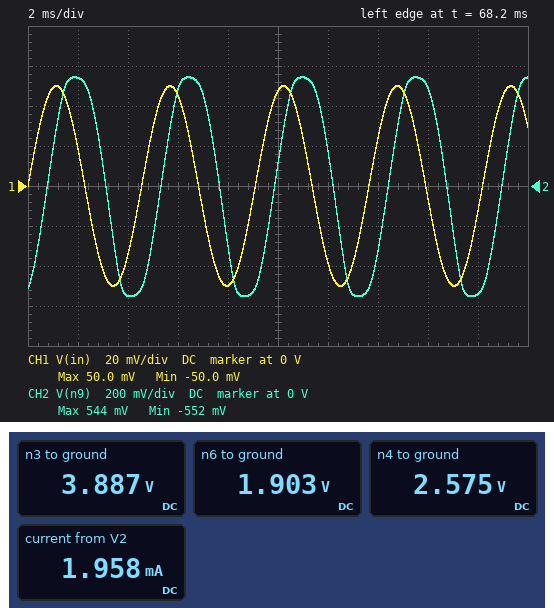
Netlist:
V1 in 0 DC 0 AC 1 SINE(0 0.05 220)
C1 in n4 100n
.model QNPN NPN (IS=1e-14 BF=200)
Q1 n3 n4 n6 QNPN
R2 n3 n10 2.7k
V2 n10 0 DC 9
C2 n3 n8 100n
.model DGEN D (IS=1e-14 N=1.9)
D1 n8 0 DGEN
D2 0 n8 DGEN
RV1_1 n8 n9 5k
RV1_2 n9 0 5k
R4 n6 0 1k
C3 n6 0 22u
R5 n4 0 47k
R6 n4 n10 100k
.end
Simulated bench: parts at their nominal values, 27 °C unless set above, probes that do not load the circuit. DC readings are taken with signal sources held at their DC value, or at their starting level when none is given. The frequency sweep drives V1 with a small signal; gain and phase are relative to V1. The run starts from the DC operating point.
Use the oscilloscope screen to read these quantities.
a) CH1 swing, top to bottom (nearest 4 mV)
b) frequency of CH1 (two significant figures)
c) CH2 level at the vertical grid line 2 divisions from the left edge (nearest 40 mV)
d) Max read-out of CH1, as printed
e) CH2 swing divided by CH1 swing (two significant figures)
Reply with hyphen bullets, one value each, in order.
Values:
- 100 mV
- 220 Hz
- -560 mV
- 50.0 mV
- 11
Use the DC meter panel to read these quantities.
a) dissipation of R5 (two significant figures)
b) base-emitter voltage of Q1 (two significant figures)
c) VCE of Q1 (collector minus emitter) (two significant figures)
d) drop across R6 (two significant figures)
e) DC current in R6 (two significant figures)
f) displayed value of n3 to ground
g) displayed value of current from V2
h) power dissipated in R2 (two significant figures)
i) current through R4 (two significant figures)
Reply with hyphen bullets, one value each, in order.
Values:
- 140 µW
- 670 mV
- 2.0 V
- 6.4 V
- 64 µA
- 3.887 V
- 1.958 mA
- 9.7 mW
- 1.9 mA
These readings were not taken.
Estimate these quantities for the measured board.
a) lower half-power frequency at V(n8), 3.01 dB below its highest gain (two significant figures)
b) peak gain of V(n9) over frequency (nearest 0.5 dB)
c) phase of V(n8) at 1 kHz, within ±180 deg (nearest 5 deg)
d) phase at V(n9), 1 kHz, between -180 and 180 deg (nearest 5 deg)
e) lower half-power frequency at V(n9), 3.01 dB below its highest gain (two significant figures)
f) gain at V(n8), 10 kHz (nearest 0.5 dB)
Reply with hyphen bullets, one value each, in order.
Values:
- 1.2 kHz
- 38.0 dB
- -125 deg
- -125 deg
- 1.2 kHz
- 44.0 dB
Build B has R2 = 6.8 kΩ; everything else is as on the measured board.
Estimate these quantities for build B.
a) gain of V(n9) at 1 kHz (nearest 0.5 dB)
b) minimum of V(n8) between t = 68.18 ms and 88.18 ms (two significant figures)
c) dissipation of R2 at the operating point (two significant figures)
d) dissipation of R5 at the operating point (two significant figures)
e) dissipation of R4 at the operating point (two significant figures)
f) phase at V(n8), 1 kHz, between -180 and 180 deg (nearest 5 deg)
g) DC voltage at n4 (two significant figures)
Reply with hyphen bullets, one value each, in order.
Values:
- -11.0 dB
- -4.9 mV
- 8.8 mW
- 71 µW
- 1.4 mW
- -80 deg
- 1.8 V
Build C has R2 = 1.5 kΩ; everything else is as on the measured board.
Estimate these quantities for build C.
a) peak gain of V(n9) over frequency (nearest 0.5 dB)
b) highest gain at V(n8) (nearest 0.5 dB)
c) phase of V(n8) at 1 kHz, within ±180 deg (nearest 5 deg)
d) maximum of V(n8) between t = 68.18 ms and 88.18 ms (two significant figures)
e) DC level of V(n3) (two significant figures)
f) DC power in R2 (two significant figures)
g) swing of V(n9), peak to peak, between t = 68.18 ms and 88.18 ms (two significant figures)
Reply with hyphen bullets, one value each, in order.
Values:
- 33.5 dB
- 39.5 dB
- -120 deg
- 730 mV
- 6.2 V
- 5.4 mW
- 750 mV
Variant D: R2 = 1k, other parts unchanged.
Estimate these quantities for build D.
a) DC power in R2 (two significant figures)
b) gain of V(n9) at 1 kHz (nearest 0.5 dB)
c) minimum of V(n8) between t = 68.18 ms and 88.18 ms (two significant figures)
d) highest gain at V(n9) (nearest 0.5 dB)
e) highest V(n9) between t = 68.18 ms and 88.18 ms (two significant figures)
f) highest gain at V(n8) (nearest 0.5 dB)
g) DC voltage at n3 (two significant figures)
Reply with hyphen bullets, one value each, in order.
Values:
- 3.6 mW
- 26.5 dB
- -540 mV
- 30.5 dB
- 250 mV
- 36.5 dB
- 7.1 V
